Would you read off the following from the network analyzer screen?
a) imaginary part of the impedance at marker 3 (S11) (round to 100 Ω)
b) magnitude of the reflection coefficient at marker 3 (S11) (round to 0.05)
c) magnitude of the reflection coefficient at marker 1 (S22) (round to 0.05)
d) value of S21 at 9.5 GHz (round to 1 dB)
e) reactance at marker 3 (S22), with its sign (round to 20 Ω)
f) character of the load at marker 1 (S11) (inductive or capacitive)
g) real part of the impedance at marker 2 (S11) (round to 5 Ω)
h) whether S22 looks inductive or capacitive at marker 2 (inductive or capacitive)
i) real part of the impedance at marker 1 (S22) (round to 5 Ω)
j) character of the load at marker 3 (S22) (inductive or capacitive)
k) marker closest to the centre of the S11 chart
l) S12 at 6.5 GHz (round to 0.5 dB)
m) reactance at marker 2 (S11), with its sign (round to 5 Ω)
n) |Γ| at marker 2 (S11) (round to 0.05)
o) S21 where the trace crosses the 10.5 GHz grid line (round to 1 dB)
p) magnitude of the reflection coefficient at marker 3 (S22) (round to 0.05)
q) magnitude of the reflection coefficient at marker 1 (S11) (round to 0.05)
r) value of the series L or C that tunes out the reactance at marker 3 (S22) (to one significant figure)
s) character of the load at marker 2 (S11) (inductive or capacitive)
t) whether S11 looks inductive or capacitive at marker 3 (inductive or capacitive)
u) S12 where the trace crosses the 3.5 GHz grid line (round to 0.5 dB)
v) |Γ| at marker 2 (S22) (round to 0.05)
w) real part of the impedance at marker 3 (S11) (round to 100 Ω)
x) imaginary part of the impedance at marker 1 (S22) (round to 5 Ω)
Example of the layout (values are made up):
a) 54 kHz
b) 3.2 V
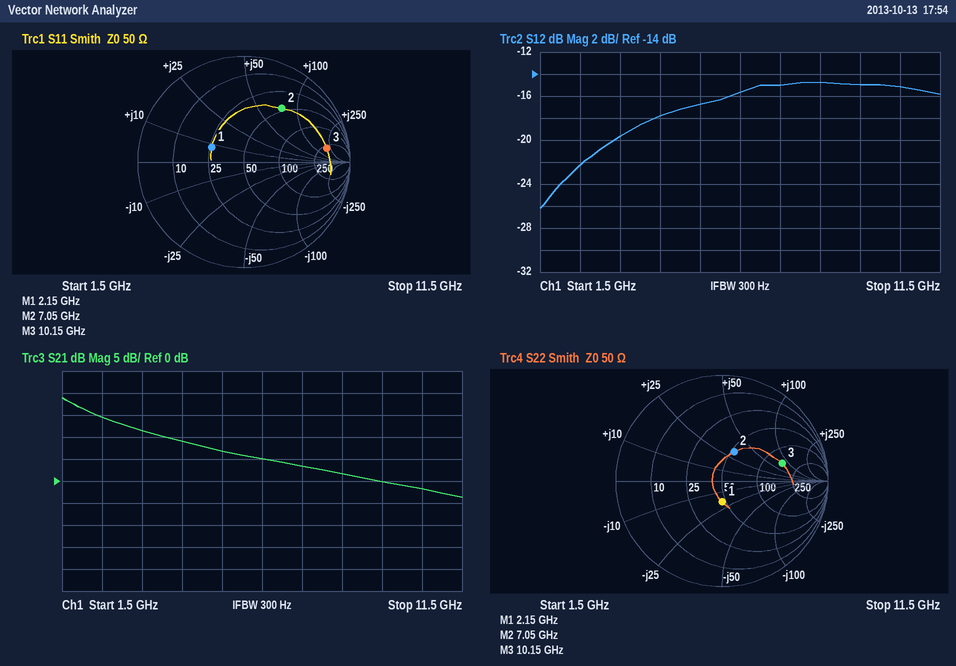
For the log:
a) +200 Ω
b) 0.80
c) 0.20
d) 0 dB
e) +80 Ω
f) inductive
g) 45 Ω
h) inductive
i) 45 Ω
j) inductive
k) marker 1
l) -15.5 dB
m) +75 Ω
n) 0.60
o) -2 dB
p) 0.60
q) 0.35
r) 200 fF
s) inductive
t) inductive
u) -19.5 dB
v) 0.30
w) 300 Ω
x) -20 Ω
